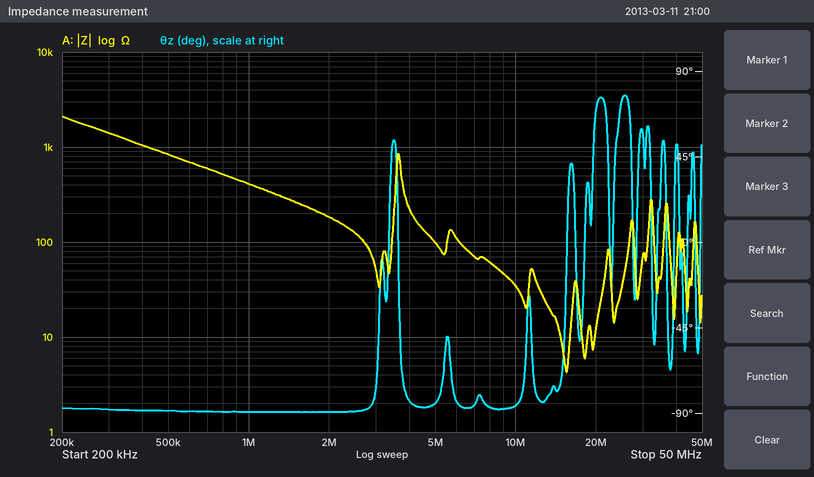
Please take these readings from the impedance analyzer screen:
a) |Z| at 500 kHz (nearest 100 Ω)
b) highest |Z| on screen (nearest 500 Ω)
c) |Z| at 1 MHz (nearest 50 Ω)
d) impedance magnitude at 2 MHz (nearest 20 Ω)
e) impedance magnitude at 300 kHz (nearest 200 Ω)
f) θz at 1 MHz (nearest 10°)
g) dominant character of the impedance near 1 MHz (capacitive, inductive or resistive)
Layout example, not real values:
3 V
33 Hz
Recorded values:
800 Ω
2.0 kΩ
400 Ω
180 Ω
1.4 kΩ
-90°
capacitive
